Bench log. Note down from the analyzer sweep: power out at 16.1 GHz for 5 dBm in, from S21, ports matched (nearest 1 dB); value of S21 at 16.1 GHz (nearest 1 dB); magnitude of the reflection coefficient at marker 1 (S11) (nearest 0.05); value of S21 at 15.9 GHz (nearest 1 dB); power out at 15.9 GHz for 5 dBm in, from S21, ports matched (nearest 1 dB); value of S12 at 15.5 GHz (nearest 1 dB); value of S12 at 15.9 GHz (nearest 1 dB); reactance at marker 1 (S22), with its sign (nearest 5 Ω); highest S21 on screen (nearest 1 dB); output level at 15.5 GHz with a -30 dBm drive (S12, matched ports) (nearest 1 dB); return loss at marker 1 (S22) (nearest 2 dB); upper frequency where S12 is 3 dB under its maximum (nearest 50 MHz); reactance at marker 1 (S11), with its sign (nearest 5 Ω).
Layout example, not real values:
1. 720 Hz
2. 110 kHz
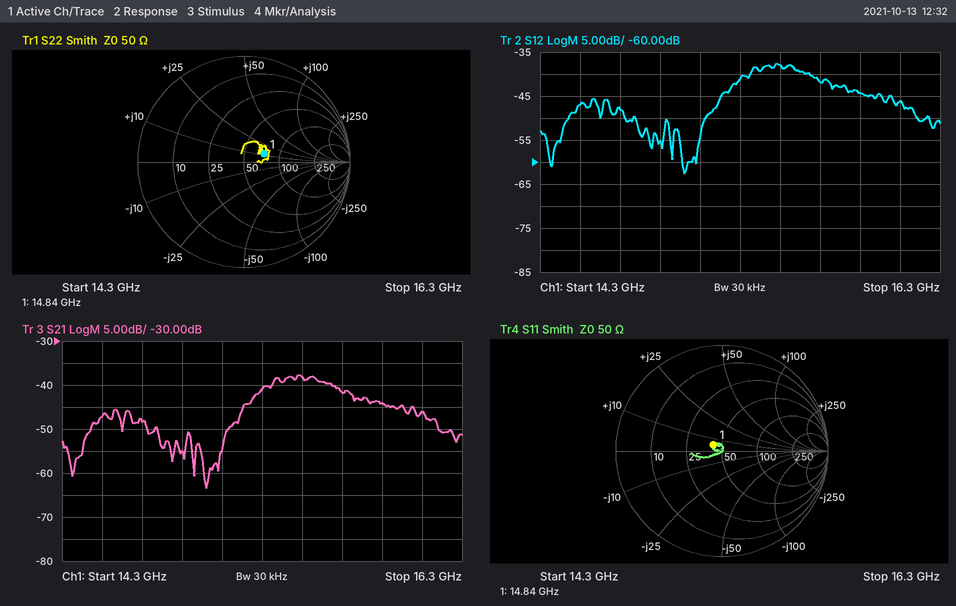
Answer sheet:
1. -41 dBm
2. -46 dB
3. 0.10
4. -44 dB
5. -39 dBm
6. -38 dB
7. -44 dB
8. +10 Ω
9. -38 dB
10. -68 dBm
11. 14 dB
12. 15.65 GHz
13. +5 Ω
